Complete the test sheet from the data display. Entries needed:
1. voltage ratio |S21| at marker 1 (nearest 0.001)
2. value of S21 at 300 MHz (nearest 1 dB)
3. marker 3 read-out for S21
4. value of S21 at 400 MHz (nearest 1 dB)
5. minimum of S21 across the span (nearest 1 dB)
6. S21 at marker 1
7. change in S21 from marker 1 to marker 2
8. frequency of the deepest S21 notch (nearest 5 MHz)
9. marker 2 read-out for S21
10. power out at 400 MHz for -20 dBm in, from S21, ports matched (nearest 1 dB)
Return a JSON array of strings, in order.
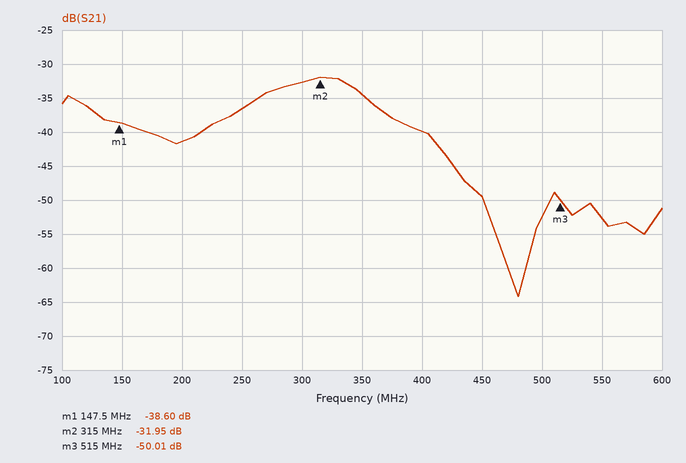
["0.012", "-33 dB", "-50.01 dB", "-40 dB", "-64 dB", "-38.60 dB", "6.65 dB", "480 MHz", "-31.95 dB", "-60 dBm"]
